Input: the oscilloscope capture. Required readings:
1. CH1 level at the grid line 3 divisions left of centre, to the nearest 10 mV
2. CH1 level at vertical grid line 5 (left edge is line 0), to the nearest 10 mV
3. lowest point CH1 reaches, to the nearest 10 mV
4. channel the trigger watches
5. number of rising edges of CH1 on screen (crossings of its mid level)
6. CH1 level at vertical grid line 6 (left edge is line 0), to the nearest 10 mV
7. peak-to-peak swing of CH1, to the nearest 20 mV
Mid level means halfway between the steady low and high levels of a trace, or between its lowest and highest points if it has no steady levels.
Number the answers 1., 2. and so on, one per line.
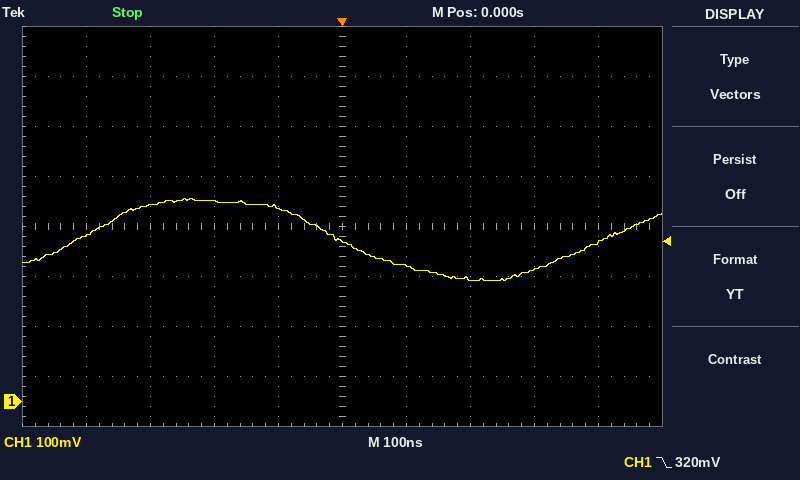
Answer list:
1. 390 mV
2. 320 mV
3. 240 mV
4. CH1
5. 2
6. 270 mV
7. 160 mV
